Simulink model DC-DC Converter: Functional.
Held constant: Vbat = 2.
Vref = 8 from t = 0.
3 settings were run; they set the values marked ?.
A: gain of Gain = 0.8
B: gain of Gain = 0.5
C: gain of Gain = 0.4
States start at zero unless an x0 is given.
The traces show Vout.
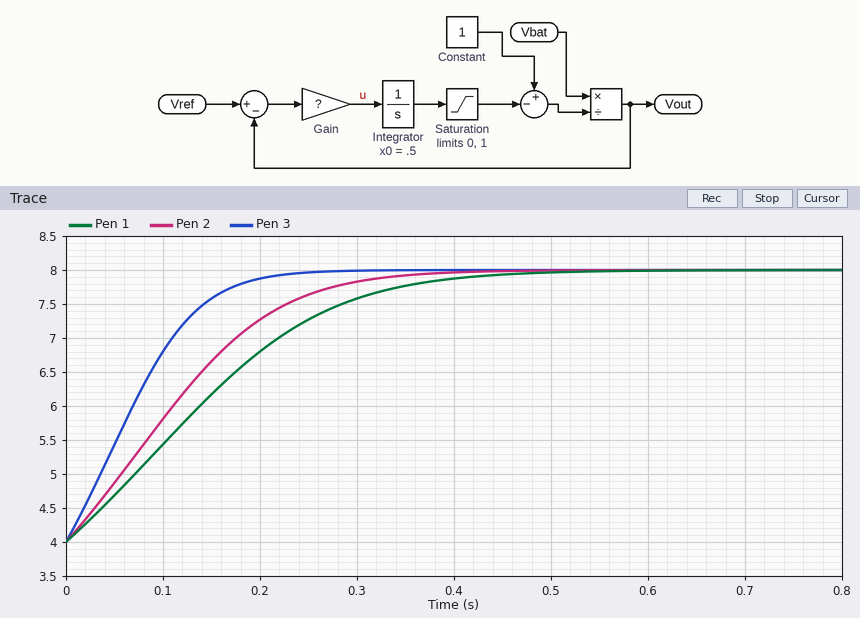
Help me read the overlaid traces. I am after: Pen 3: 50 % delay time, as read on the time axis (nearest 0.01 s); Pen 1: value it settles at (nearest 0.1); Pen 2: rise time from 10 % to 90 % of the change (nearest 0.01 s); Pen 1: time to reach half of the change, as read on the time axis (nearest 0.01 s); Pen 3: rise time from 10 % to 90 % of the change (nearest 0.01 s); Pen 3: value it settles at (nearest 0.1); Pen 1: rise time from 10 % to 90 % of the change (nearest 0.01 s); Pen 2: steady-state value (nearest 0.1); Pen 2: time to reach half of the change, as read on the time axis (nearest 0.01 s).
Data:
0.07 s
8.0
0.22 s
0.14 s
0.14 s
8.0
0.27 s
8.0
0.11 s
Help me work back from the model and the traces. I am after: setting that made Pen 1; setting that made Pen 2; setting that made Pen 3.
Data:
C
B
A
